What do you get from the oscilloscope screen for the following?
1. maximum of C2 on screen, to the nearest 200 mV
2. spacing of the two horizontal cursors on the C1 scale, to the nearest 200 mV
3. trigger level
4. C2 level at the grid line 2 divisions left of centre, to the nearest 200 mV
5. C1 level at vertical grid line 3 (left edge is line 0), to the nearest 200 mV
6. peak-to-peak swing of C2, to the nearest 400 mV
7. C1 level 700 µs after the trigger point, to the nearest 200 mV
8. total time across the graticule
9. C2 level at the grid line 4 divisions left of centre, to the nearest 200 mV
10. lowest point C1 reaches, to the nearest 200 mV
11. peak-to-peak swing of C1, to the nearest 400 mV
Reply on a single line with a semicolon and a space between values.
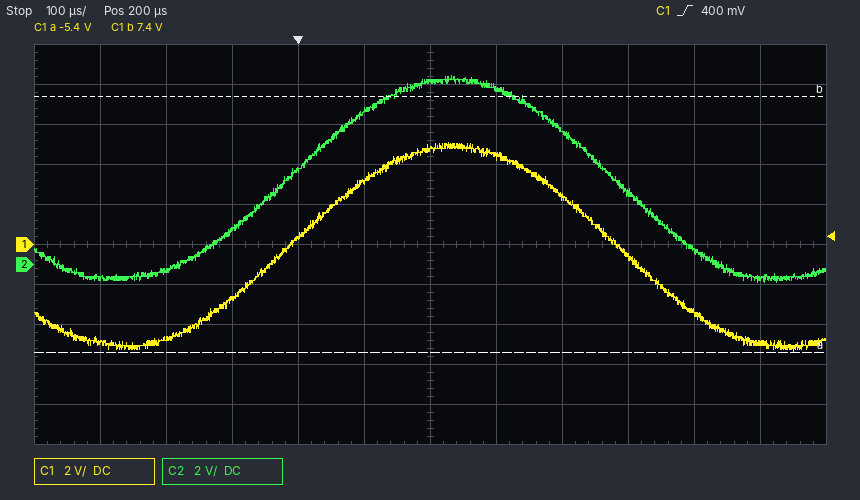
9.4 V; 12.8 V; 400 mV; 4.8 V; -2.8 V; 10.4 V; -5.0 V; 1.2 ms; -400 mV; -5.4 V; 10.4 V
